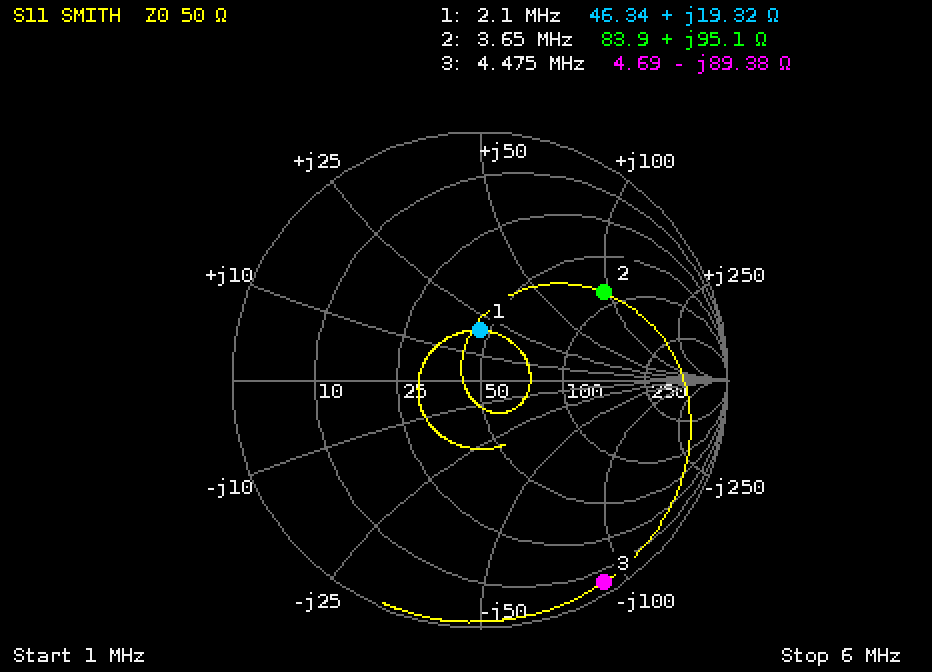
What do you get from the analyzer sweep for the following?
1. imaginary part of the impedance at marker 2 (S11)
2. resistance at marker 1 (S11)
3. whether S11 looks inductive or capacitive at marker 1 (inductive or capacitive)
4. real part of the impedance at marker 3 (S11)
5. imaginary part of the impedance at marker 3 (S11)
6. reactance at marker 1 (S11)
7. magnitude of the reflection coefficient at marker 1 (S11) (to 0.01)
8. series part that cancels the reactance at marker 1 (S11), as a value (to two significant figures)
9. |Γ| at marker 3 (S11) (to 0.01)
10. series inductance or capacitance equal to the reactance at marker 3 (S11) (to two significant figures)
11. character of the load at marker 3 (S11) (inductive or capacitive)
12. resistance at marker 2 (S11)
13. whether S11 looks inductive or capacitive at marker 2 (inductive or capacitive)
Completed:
+95.1 Ω
46.34 Ω
inductive
4.69 Ω
-89.38 Ω
+19.32 Ω
0.20
3.9 nF
0.96
400 pF
capacitive
83.9 Ω
inductive
